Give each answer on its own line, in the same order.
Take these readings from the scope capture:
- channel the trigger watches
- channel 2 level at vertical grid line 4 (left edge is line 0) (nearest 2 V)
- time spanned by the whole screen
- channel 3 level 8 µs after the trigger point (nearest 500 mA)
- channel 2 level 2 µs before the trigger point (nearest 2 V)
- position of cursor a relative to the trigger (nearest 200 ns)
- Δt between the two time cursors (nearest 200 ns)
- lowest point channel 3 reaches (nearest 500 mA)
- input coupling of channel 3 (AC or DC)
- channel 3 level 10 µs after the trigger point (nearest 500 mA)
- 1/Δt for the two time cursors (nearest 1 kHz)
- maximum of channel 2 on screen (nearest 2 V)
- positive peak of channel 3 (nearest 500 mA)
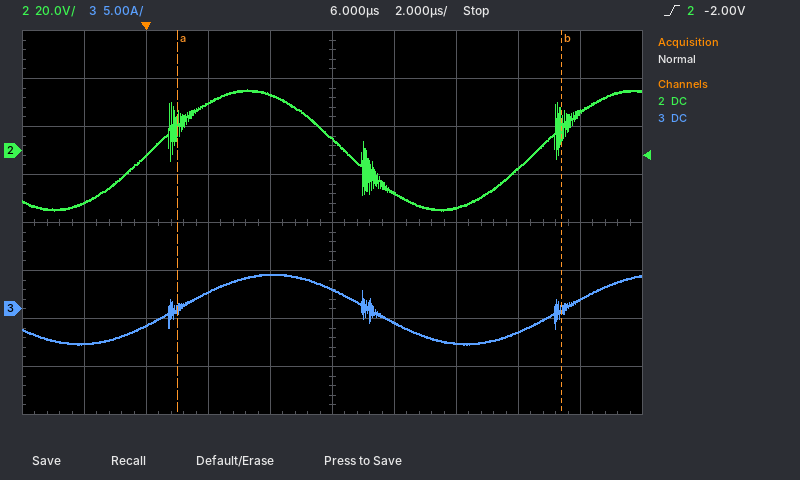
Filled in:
channel 2
24 V
20 µs
-1.5 A
-22 V
+1.0 µs
12.4 µs
-3.5 A
DC
-3.5 A
81 kHz
26 V
3.5 A
